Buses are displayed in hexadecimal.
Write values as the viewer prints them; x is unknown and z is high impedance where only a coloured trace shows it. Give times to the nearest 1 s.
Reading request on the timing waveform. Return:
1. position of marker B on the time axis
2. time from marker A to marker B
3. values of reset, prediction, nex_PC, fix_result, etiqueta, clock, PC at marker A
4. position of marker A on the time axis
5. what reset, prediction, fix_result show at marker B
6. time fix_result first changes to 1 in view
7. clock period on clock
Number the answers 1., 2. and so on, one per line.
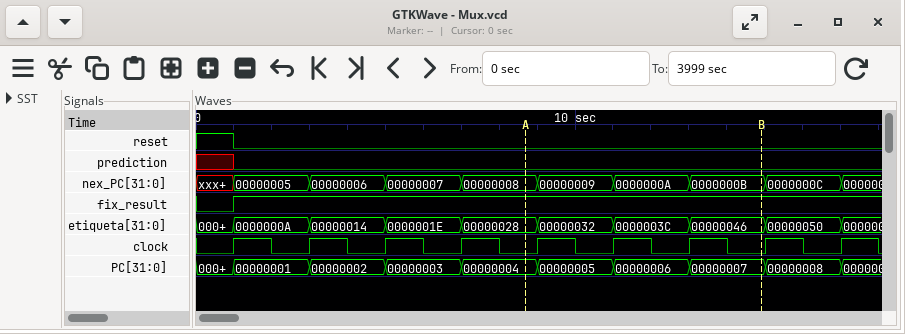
1. 15 s
2. 6 s
3. reset=0, prediction=0, nex_PC=00000008, fix_result=1, etiqueta=00000028, clock=0, PC=00000004
4. 9 s
5. reset=0, prediction=0, fix_result=1
6. 1 s
7. 2 s
